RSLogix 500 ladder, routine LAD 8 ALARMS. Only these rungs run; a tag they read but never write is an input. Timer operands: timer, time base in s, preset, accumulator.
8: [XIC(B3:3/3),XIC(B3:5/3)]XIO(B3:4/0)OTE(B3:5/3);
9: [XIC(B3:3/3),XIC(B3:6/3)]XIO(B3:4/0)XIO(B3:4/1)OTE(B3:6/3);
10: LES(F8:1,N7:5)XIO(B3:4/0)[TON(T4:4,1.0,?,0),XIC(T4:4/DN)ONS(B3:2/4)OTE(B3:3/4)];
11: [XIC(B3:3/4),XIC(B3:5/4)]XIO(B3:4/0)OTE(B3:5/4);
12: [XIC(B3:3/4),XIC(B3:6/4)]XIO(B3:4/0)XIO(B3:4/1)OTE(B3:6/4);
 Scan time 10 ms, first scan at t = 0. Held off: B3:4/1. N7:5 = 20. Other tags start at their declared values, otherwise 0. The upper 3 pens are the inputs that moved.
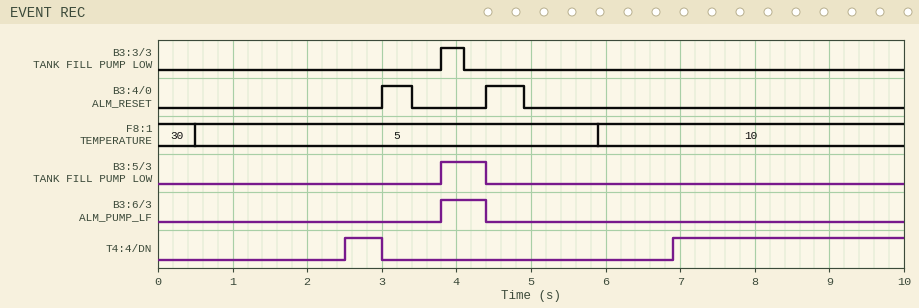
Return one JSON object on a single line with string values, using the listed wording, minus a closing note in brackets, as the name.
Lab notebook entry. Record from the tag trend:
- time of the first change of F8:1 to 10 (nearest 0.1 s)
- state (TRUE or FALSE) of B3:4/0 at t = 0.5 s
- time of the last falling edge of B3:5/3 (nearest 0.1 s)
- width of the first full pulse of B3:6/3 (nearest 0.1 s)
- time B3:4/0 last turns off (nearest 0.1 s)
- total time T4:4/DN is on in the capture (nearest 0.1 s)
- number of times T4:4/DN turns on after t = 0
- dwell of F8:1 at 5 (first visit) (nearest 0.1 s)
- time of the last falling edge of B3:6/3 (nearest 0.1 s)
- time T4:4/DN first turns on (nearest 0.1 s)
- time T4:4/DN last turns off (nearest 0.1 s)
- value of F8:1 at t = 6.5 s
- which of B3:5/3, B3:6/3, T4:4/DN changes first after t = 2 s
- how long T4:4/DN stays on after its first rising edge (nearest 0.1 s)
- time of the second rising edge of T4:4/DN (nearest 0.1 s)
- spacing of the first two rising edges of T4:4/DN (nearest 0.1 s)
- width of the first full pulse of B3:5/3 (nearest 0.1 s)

{"time of the first change of F8:1 to 10": "5.9 s", "state (TRUE or FALSE) of B3:4/0 at t = 0.5 s": "FALSE", "time of the last falling edge of B3:5/3": "4.4 s", "width of the first full pulse of B3:6/3": "0.6 s", "time B3:4/0 last turns off": "4.9 s", "total time T4:4/DN is on in the capture": "3.6 s", "number of times T4:4/DN turns on after t = 0": "2", "dwell of F8:1 at 5 (first visit)": "5.4 s", "time of the last falling edge of B3:6/3": "4.4 s", "time T4:4/DN first turns on": "2.5 s", "time T4:4/DN last turns off": "3.0 s", "value of F8:1 at t = 6.5 s": "10", "which of B3:5/3, B3:6/3, T4:4/DN changes first after t = 2 s": "T4:4/DN", "how long T4:4/DN stays on after its first rising edge": "0.5 s", "time of the second rising edge of T4:4/DN": "6.9 s", "spacing of the first two rising edges of T4:4/DN": "4.4 s", "width of the first full pulse of B3:5/3": "0.6 s"}
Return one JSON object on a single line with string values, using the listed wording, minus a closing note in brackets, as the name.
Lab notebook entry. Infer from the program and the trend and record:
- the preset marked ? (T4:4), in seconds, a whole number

{"the preset marked ? (T4:4), in seconds, a whole number": "2 s"}
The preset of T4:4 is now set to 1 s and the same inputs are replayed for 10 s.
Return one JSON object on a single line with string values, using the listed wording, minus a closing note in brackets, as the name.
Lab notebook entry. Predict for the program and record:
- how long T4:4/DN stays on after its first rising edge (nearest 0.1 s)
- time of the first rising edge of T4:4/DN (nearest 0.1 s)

{"how long T4:4/DN stays on after its first rising edge": "1.5 s", "time of the first rising edge of T4:4/DN": "1.5 s"}
